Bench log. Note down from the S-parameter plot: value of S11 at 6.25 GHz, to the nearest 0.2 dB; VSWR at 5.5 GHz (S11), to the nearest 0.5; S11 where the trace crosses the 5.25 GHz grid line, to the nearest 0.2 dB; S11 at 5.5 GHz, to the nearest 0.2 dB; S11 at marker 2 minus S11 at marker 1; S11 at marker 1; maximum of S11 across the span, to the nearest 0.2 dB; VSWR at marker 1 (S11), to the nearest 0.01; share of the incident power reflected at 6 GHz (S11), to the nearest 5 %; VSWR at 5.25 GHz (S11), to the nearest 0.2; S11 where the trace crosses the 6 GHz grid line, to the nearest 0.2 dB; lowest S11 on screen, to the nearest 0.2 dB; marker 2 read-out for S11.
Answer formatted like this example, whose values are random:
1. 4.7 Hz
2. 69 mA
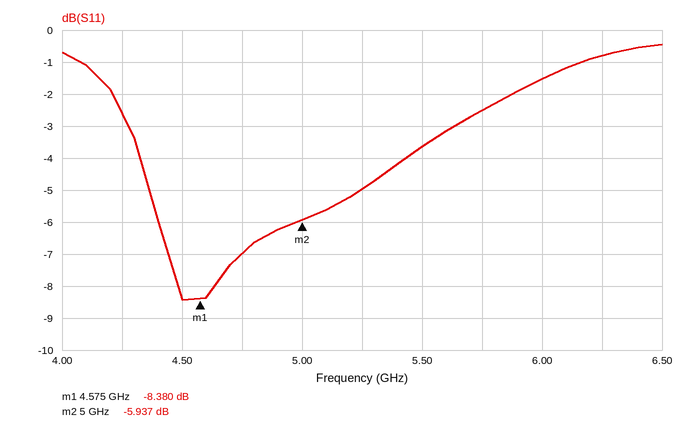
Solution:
1. -0.8 dB
2. 5.0
3. -5.0 dB
4. -3.6 dB
5. 2.443 dB
6. -8.380 dB
7. -0.4 dB
8. 2.23
9. 70 %
10. 3.6
11. -1.6 dB
12. -8.4 dB
13. -5.937 dB
